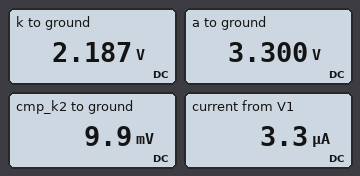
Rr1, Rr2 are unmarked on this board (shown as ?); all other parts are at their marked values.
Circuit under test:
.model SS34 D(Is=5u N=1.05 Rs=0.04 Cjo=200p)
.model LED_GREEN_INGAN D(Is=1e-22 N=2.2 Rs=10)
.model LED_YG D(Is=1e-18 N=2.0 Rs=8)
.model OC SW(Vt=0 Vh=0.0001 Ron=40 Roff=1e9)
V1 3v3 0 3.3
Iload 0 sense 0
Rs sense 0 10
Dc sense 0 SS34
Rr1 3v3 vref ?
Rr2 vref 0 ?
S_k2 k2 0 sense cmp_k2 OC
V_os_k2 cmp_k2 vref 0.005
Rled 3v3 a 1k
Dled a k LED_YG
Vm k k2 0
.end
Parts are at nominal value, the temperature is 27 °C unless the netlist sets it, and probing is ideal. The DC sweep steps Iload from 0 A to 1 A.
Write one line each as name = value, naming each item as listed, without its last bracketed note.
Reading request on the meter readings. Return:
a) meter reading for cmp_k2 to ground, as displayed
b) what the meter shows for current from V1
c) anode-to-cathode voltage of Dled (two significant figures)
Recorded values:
meter reading for cmp_k2 to ground, as displayed = 9.9 mV
what the meter shows for current from V1 = 3.3 µA
anode-to-cathode voltage of Dled = 1.1 V
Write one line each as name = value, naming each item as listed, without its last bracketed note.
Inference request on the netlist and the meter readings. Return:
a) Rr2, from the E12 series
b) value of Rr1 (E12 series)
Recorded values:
Rr2, from the E12 series = 1.5 kΩ
value of Rr1 = 1 MΩ
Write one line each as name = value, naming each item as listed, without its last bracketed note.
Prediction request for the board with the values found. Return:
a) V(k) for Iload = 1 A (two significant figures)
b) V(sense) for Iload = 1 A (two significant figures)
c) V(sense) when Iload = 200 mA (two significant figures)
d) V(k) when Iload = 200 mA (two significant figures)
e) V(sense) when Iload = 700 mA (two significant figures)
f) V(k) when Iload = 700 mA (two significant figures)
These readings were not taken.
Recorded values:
V(k) for Iload = 1 A = 57 mV
V(sense) for Iload = 1 A = 370 mV
V(sense) when Iload = 200 mA = 290 mV
V(k) when Iload = 200 mA = 57 mV
V(sense) when Iload = 700 mA = 350 mV
V(k) when Iload = 700 mA = 57 mV
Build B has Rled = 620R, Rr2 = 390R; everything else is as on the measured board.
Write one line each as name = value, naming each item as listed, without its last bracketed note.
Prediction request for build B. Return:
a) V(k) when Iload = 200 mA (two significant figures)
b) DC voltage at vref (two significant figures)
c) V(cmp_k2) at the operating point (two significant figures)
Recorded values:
V(k) when Iload = 200 mA = 88 mV
DC voltage at vref = 1.3 mV
V(cmp_k2) at the operating point = 6.3 mV
